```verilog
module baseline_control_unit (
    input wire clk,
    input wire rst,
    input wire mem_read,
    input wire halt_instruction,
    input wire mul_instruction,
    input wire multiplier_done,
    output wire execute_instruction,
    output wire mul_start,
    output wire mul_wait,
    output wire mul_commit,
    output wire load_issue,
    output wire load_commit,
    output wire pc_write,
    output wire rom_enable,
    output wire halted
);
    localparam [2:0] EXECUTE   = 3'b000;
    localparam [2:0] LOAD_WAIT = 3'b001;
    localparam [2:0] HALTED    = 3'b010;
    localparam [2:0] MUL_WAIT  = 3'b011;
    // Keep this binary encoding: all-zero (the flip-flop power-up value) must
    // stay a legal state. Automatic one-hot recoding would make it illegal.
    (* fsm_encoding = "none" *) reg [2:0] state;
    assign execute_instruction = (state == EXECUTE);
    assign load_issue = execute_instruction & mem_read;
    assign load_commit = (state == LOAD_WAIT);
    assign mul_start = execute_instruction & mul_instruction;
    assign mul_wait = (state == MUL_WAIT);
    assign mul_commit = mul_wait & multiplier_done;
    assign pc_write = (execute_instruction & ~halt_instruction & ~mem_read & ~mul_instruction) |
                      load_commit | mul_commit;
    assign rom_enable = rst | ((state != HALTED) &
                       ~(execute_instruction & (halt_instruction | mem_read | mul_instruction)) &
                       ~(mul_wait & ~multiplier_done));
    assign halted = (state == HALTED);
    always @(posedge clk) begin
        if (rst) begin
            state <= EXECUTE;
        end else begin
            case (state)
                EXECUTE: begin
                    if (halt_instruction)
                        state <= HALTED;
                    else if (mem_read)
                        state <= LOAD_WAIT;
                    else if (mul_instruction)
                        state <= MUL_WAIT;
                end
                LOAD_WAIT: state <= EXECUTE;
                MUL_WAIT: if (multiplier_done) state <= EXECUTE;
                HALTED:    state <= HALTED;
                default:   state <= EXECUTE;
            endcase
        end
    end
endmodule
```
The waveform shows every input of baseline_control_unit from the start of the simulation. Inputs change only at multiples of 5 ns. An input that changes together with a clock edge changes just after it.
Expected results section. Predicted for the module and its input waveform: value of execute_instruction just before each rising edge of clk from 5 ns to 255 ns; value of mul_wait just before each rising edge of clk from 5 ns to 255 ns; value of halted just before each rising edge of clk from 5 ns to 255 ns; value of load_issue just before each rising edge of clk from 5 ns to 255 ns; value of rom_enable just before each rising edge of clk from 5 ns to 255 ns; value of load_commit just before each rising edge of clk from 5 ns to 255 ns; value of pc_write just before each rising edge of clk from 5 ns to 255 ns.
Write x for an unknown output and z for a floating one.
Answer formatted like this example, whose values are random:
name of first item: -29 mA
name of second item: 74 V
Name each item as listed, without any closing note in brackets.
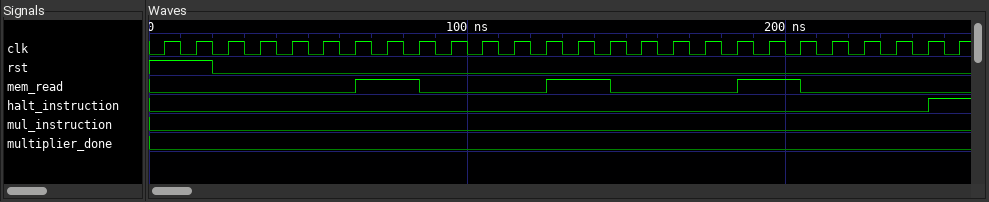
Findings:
value of execute_instruction just before each rising edge of clk from 5 ns to 255 ns: x 1 1 1 1 1 1 1 0 1 1 1 1 1 0 1 1 1 1 1 0 1 1 1 1 1
value of mul_wait just before each rising edge of clk from 5 ns to 255 ns: x 0 0 0 0 0 0 0 0 0 0 0 0 0 0 0 0 0 0 0 0 0 0 0 0 0
value of halted just before each rising edge of clk from 5 ns to 255 ns: x 0 0 0 0 0 0 0 0 0 0 0 0 0 0 0 0 0 0 0 0 0 0 0 0 0
value of load_issue just before each rising edge of clk from 5 ns to 255 ns: 0 0 0 0 0 0 0 1 0 0 0 0 0 1 0 0 0 0 0 1 0 0 0 0 0 0
value of rom_enable just before each rising edge of clk from 5 ns to 255 ns: 1 1 1 1 1 1 1 0 1 1 1 1 1 0 1 1 1 1 1 0 1 1 1 1 1 0
value of load_commit just before each rising edge of clk from 5 ns to 255 ns: x 0 0 0 0 0 0 0 1 0 0 0 0 0 1 0 0 0 0 0 1 0 0 0 0 0
value of pc_write just before each rising edge of clk from 5 ns to 255 ns: x 1 1 1 1 1 1 0 1 1 1 1 1 0 1 1 1 1 1 0 1 1 1 1 1 0
